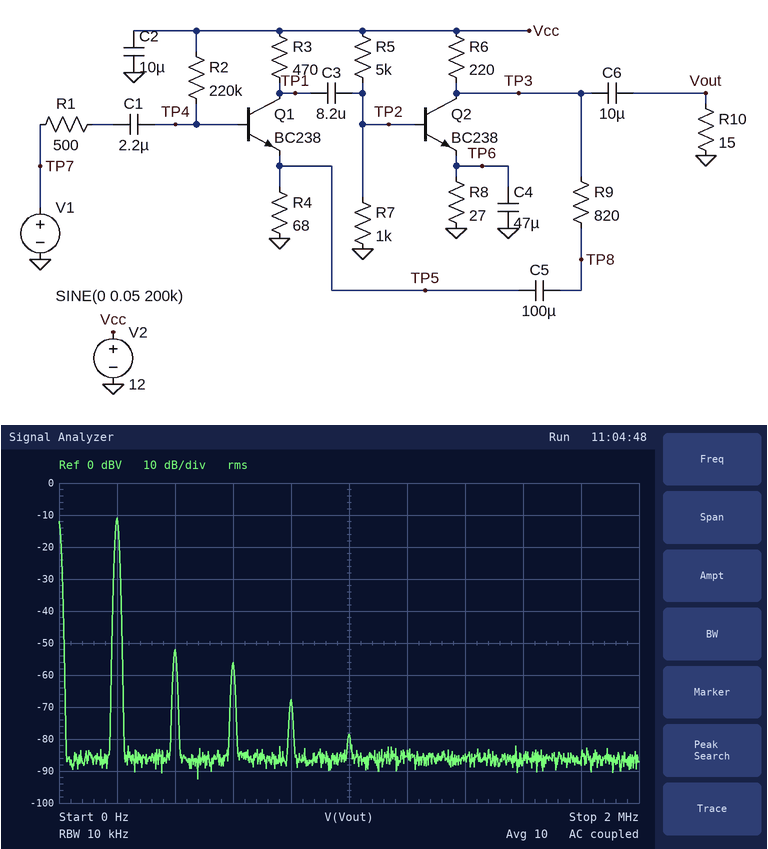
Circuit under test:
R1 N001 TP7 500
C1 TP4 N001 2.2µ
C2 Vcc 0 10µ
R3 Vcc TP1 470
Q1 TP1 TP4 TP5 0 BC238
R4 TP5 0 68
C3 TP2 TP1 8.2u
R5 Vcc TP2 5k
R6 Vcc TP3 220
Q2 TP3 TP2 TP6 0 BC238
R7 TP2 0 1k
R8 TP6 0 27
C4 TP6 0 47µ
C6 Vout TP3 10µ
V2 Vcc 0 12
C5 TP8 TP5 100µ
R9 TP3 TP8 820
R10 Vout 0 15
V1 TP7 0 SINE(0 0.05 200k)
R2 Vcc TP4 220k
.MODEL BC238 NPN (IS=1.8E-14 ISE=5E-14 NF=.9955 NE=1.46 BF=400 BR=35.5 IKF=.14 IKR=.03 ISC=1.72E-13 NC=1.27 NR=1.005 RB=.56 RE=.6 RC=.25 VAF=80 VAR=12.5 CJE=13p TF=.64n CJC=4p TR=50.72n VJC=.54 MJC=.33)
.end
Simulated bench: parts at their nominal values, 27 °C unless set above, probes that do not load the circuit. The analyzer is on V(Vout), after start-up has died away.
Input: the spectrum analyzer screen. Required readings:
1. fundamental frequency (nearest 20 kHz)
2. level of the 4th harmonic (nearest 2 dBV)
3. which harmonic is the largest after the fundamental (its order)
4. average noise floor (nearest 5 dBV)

200 kHz
-68 dBV
2
-85 dBV
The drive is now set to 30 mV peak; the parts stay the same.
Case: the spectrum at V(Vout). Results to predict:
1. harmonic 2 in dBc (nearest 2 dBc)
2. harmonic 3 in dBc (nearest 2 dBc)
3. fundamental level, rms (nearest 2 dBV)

-50 dBc
-56 dBc
-16 dBV
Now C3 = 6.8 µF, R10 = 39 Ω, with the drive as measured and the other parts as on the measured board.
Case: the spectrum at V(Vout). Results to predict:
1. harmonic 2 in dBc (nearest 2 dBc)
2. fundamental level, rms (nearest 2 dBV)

-58 dBc
-8 dBV
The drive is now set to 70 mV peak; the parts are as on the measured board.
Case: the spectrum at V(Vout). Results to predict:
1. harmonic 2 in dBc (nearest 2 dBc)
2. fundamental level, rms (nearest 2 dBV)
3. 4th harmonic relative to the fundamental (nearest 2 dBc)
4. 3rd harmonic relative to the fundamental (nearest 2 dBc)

-32 dBc
-8 dBV
-44 dBc
-36 dBc
